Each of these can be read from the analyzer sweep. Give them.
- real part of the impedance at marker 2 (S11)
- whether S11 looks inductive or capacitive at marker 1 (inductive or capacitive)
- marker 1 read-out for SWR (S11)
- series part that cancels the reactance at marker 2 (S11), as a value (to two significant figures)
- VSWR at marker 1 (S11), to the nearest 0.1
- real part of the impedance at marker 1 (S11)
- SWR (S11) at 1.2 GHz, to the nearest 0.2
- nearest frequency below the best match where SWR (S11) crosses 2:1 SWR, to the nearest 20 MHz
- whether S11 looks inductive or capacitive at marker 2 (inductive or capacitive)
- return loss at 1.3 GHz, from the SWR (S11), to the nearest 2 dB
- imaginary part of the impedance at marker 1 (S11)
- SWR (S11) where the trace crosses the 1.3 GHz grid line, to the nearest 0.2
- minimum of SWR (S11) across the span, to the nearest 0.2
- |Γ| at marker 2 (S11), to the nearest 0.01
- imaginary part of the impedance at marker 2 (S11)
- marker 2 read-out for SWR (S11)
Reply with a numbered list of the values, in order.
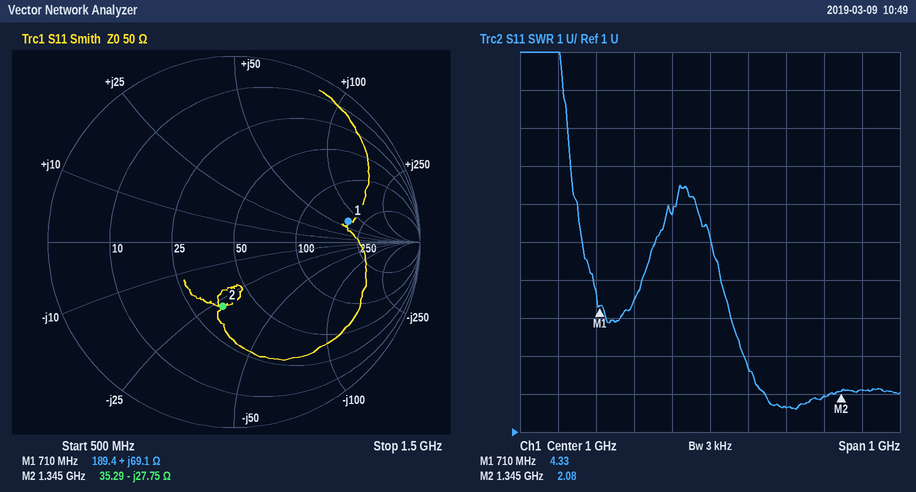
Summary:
1. 35.29 Ω
2. inductive
3. 4.33
4. 3.3 nH
5. 4.3
6. 189.4 Ω
7. 1.6
8. 1.14 GHz
9. capacitive
10. 10 dB
11. +69.1 Ω
12. 2.0
13. 1.6
14. 0.35
15. -27.75 Ω
16. 2.08
